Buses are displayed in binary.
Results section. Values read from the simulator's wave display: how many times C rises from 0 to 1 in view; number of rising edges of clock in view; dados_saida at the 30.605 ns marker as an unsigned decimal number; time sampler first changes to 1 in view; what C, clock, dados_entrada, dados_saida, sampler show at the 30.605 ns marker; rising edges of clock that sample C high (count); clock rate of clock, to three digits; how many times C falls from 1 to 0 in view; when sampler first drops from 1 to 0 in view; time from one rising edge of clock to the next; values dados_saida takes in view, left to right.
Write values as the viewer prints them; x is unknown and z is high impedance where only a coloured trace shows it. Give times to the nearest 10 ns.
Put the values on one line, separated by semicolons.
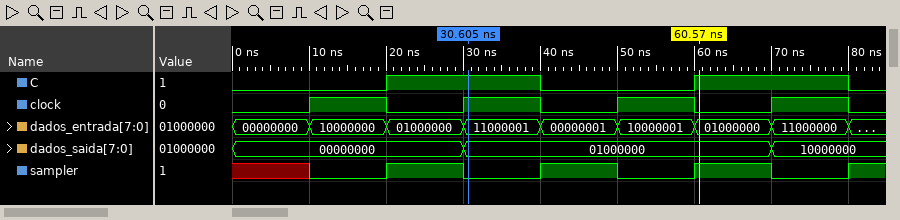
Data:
2; 4; 64; 20 ns; C=1, clock=1, dados_entrada=11000001, dados_saida=01000000, sampler=0; 2; 50.0 MHz; 2; 30 ns; 20 ns; 00000000, 01000000, 10000000
